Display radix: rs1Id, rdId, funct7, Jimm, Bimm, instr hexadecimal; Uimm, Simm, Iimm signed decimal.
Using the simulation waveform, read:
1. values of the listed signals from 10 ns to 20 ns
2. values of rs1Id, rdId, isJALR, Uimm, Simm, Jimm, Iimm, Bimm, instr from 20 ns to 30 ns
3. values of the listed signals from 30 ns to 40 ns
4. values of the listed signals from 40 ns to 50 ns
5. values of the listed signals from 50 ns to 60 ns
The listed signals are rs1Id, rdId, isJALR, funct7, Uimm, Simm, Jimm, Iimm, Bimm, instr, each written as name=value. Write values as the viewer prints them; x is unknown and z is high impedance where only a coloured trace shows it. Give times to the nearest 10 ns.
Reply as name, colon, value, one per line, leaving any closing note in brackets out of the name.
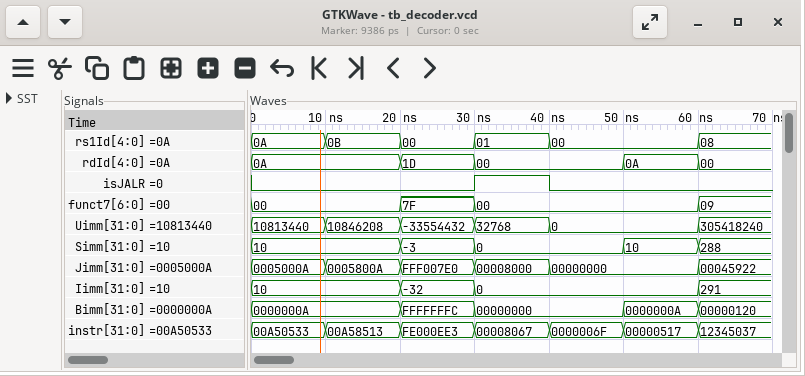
values of the listed signals from 10 ns to 20 ns: rs1Id=0B, rdId=0A, isJALR=0, funct7=00, Uimm=10846208, Simm=10, Jimm=0005800A, Iimm=10, Bimm=0000000A, instr=00A58513
values of rs1Id, rdId, isJALR, Uimm, Simm, Jimm, Iimm, Bimm, instr from 20 ns to 30 ns: rs1Id=00, rdId=1D, isJALR=0, Uimm=-33554432, Simm=-3, Jimm=FFF007E0, Iimm=-32, Bimm=FFFFFFFC, instr=FE000EE3
values of the listed signals from 30 ns to 40 ns: rs1Id=01, rdId=00, isJALR=1, funct7=00, Uimm=32768, Simm=0, Jimm=00008000, Iimm=0, Bimm=00000000, instr=00008067
values of the listed signals from 40 ns to 50 ns: rs1Id=00, rdId=00, isJALR=0, funct7=00, Uimm=0, Simm=0, Jimm=00000000, Iimm=0, Bimm=00000000, instr=0000006F
values of the listed signals from 50 ns to 60 ns: rs1Id=00, rdId=0A, isJALR=0, funct7=00, Uimm=0, Simm=10, Jimm=00000000, Iimm=0, Bimm=0000000A, instr=00000517
